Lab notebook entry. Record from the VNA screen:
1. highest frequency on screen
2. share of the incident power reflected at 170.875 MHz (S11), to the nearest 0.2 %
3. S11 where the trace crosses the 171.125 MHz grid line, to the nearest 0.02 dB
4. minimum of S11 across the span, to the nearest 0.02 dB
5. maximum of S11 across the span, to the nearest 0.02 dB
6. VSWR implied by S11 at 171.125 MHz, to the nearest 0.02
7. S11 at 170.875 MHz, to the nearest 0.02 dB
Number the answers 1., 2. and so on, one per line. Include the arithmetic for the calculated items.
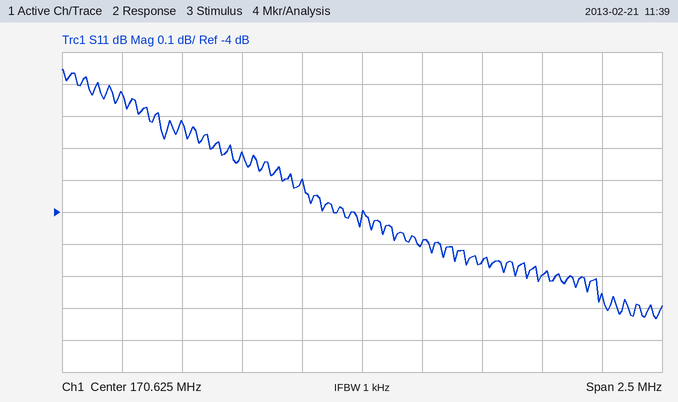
1. 171.875 MHz
2. 10^(-4.1/10) ≈ 38.9 %, so 39.0 % to the nearest 0.2 %
3. -4.16 dB
4. -4.34 dB
5. -3.56 dB
6. |Γ| = 10^(-4.16/20) = 0.6194; VSWR = (1 + 0.6194)/(1 − 0.6194) ≈ 4.26
7. -4.10 dB
